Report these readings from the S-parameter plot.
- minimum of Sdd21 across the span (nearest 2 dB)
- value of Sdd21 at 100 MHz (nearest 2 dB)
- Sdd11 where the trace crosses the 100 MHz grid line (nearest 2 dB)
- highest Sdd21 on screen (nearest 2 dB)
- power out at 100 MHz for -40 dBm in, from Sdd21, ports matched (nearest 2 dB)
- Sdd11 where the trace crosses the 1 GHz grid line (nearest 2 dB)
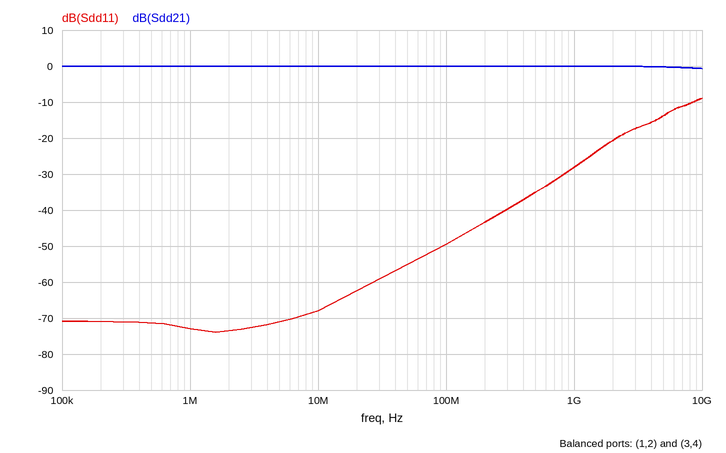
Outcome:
0 dB
0 dB
-50 dB
0 dB
-40 dBm
-28 dB
